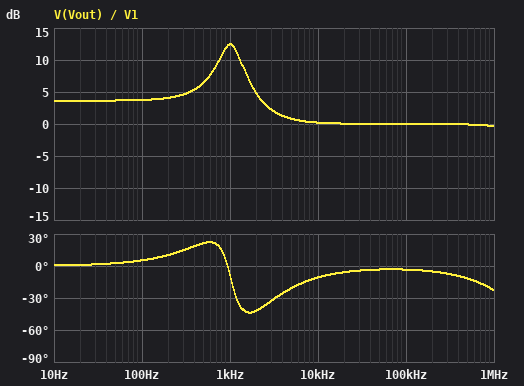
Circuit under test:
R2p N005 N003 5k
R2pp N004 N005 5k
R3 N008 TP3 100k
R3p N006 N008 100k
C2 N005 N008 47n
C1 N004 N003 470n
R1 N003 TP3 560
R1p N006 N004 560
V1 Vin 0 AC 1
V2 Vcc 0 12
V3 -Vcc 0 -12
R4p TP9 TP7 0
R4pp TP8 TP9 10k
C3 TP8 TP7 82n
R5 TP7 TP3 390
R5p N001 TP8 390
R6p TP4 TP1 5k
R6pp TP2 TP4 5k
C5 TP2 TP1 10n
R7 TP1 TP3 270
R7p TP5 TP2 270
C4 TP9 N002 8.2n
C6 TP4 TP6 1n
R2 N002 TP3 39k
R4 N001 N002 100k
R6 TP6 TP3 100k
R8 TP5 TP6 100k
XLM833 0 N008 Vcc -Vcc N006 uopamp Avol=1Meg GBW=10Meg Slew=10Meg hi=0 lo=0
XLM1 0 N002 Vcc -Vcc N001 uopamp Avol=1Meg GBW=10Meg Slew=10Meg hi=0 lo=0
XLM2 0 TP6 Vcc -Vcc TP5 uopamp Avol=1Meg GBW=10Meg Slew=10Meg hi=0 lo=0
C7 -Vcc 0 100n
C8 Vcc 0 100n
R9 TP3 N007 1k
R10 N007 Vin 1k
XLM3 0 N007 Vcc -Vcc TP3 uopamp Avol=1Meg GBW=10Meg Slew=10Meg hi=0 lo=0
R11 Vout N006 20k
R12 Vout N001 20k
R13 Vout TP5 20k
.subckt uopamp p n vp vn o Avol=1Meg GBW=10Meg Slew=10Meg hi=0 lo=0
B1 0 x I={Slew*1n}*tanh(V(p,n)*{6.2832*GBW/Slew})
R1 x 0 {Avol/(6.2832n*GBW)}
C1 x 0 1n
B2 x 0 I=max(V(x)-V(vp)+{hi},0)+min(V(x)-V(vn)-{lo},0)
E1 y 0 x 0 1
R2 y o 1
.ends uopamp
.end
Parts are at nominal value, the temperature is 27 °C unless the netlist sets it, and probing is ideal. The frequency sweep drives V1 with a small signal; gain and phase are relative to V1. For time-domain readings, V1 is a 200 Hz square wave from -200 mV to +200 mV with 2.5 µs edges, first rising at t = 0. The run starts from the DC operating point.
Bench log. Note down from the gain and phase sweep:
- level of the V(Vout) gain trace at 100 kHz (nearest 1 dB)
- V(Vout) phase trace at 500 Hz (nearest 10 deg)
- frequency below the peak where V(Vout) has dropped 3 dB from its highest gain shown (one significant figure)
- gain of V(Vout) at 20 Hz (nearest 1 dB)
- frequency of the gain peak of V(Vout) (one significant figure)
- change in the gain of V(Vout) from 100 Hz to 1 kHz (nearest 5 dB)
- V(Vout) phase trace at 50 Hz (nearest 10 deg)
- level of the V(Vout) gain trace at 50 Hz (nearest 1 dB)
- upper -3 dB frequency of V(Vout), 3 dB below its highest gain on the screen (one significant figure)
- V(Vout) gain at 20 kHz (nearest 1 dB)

0 dB
20 deg
700 Hz
4 dB
1 kHz
10 dB
0 deg
4 dB
1 kHz
0 dB
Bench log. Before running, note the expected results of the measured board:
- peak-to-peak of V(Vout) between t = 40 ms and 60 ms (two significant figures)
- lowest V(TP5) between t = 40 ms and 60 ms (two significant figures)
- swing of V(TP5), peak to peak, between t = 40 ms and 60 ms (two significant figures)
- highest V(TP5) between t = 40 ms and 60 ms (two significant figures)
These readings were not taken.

1.5 V
-200 mV
400 mV
200 mV
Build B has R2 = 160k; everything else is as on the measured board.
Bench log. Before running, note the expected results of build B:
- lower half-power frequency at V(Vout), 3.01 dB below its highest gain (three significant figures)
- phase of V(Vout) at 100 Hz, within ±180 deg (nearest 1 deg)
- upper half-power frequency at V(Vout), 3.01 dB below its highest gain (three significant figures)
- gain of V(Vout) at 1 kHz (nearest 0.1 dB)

770 Hz
10 deg
1.44 kHz
11.2 dB
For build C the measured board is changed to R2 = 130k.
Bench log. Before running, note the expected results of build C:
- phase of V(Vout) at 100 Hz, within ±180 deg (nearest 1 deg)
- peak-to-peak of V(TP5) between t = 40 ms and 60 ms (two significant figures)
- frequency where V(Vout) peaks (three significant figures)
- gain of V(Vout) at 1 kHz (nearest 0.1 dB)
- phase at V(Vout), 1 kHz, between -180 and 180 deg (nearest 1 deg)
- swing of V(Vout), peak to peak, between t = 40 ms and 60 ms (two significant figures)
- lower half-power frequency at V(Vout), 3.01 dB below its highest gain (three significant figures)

9 deg
400 mV
1.03 kHz
11.3 dB
6 deg
1.3 V
766 Hz
